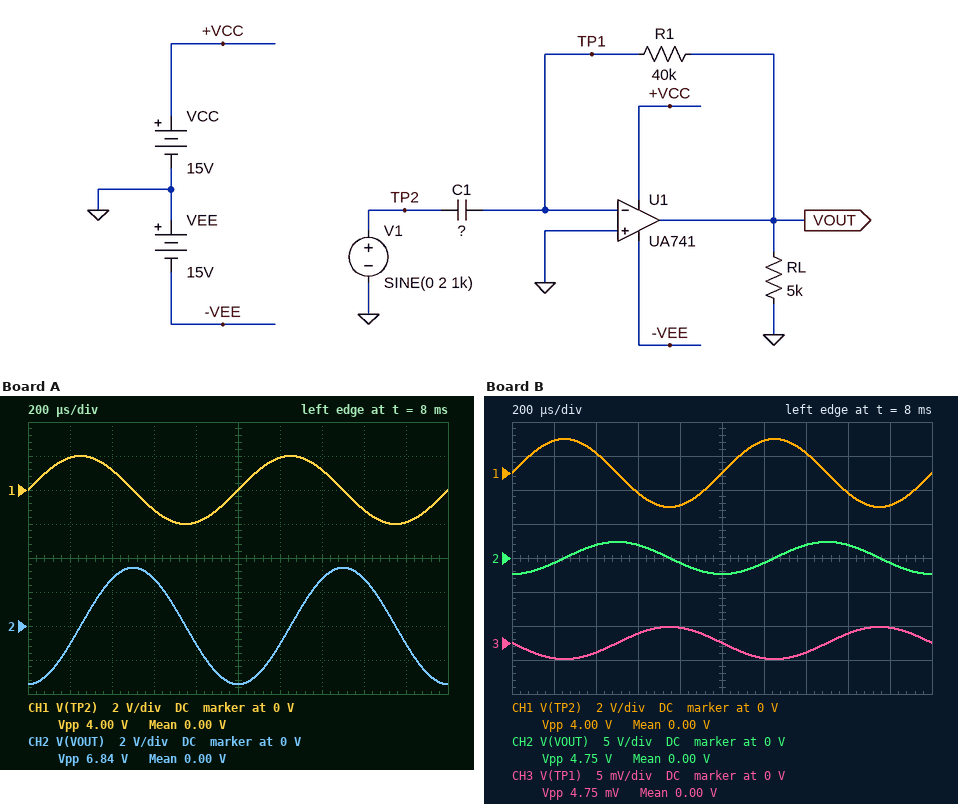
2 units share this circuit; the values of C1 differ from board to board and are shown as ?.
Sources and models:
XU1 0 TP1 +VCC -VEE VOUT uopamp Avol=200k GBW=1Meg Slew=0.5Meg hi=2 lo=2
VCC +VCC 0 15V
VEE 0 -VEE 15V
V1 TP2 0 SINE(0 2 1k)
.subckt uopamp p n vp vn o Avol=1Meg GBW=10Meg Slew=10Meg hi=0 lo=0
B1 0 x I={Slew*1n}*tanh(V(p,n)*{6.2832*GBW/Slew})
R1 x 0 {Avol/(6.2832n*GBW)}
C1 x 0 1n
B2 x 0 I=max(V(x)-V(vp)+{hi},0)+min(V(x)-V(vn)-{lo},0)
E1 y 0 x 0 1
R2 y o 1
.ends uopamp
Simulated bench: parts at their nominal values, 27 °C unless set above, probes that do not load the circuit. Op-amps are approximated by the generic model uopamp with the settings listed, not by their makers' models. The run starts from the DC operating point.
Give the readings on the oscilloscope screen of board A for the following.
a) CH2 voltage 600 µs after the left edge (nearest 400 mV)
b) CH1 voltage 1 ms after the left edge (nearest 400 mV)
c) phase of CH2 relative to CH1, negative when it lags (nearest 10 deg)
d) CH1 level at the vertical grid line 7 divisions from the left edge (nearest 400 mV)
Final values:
2.8 V
0 V
-90 deg
1.2 V
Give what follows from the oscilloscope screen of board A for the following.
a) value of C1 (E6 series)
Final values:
6.8 nF
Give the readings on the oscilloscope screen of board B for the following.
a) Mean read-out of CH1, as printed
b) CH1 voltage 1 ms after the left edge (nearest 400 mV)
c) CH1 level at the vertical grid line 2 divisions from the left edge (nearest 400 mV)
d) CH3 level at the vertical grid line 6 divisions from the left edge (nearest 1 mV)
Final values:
0.00 V
0 V
1.2 V
-2 mV
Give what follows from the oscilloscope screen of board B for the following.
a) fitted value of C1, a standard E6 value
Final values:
4.7 nF
